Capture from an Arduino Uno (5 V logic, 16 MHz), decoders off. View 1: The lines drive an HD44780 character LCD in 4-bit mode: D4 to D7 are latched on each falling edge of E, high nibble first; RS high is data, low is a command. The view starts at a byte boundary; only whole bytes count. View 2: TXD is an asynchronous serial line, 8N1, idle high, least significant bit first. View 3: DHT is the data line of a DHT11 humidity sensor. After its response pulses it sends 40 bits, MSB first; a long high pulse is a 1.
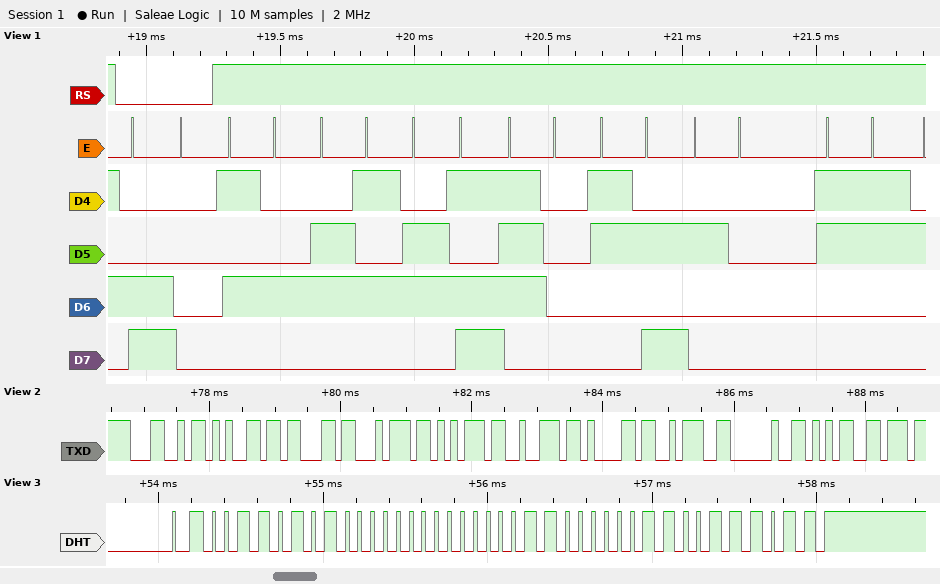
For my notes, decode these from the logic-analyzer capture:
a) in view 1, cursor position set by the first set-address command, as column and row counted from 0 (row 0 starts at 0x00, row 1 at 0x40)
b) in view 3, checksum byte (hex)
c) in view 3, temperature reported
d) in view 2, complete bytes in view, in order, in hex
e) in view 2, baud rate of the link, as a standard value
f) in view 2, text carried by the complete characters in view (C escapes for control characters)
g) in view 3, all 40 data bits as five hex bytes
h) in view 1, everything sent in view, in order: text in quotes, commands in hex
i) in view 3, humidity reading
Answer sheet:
column 0, row 1
0x3B
3.3 °C
4C 65 63 74 75 72 61 3A 20 35
9600 baud
"Lectura: 5"
35 00 03 03 3B
0xC0 "Temp: 3"
53 %
